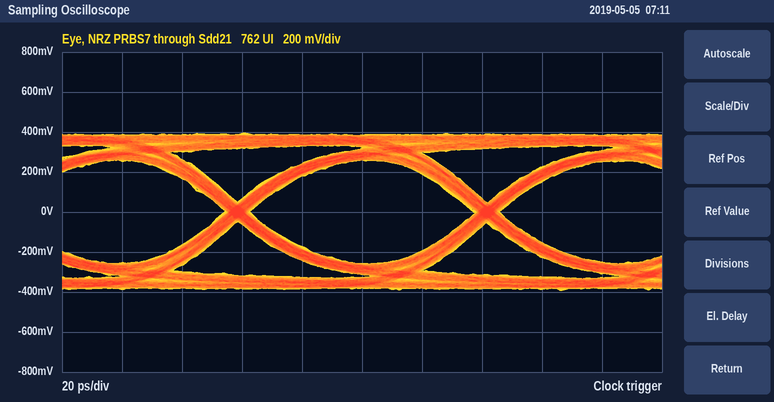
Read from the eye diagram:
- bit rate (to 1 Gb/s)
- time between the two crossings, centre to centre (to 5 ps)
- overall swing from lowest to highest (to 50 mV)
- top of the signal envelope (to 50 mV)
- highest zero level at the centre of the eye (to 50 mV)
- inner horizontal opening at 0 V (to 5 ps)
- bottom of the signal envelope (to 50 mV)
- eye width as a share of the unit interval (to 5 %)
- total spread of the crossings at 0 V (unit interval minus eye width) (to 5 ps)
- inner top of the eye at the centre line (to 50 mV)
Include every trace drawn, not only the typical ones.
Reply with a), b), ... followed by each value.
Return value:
a) 12 Gb/s
b) 85 ps
c) 800 mV
d) 400 mV
e) -250 mV
f) 75 ps
g) -400 mV
h) 90 %
i) 10 ps
j) 250 mV
